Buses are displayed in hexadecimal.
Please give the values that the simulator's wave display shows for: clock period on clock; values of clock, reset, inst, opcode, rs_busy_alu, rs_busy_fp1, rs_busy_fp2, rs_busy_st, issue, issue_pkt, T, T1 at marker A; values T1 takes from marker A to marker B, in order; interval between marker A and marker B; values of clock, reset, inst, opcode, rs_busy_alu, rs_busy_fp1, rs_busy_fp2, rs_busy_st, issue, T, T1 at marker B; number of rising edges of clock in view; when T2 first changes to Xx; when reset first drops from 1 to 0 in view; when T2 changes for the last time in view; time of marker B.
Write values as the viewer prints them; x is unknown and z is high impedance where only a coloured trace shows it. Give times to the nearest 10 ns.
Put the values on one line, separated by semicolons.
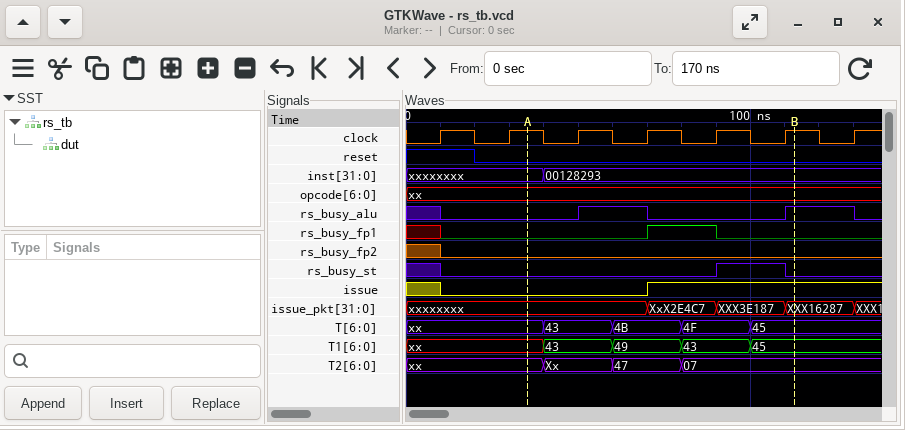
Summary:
20 ns; clock=1, reset=0, inst=xxxxxxxx, opcode=xx, rs_busy_alu=0, rs_busy_fp1=0, rs_busy_fp2=0, rs_busy_st=0, issue=0, issue_pkt=xxxxxxxx, T=xx, T1=xx; xx, 43, 49, 43, 45; 80 ns; clock=1, reset=0, inst=00128293, opcode=xx, rs_busy_alu=1, rs_busy_fp1=0, rs_busy_fp2=0, rs_busy_st=0, issue=1, T=45, T1=45; 7; 40 ns; 20 ns; 80 ns; 110 ns
